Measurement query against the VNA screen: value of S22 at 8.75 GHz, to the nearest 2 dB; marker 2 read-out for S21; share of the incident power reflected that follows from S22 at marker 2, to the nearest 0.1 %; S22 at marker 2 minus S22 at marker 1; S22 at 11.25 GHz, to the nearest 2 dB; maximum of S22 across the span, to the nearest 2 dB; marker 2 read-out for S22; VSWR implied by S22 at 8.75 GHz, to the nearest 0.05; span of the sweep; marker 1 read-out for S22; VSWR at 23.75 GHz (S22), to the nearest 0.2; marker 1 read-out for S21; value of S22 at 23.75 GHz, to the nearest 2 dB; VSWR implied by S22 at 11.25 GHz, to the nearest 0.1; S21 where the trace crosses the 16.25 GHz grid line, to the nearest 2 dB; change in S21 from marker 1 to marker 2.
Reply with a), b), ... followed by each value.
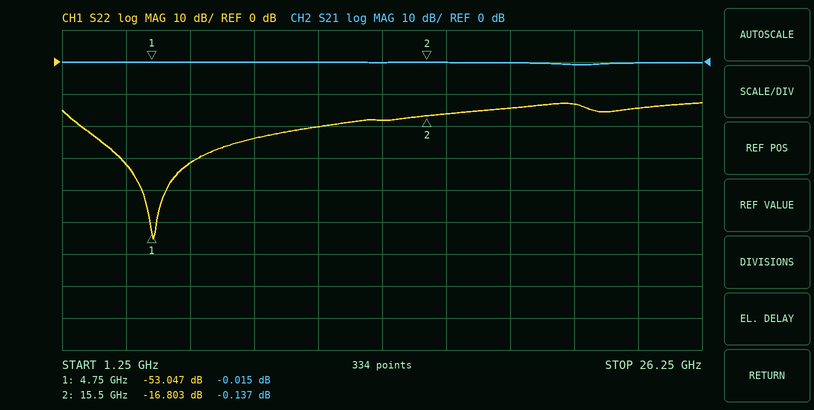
a) -24 dB
b) -0.137 dB
c) 2.1 %
d) 36.244 dB
e) -20 dB
f) -12 dB
g) -16.803 dB
h) 1.15
i) 25 GHz
j) -53.047 dB
k) 1.4
l) -0.015 dB
m) -14 dB
n) 1.2
o) 0 dB
p) -0.122 dB
